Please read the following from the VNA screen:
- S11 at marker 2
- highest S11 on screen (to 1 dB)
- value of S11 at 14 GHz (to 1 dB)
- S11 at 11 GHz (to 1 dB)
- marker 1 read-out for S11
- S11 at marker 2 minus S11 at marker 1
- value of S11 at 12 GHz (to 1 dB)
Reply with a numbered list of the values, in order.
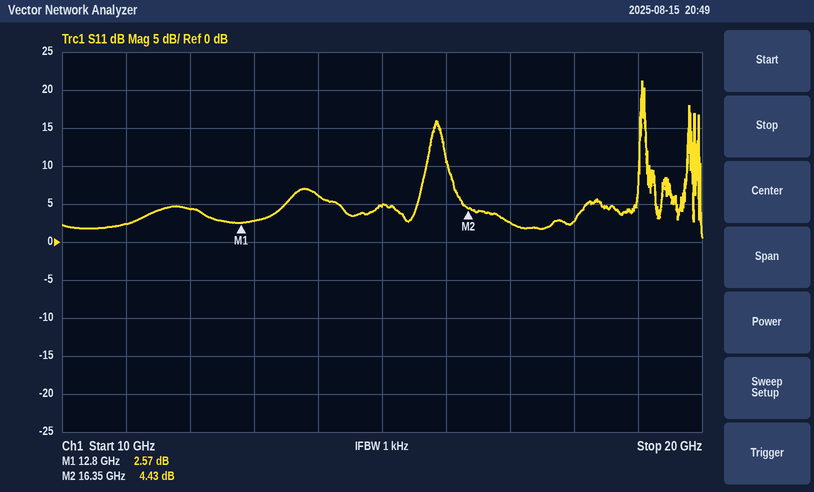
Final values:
1. 4.43 dB
2. 21 dB
3. 6 dB
4. 2 dB
5. 2.57 dB
6. 1.86 dB
7. 4 dB
